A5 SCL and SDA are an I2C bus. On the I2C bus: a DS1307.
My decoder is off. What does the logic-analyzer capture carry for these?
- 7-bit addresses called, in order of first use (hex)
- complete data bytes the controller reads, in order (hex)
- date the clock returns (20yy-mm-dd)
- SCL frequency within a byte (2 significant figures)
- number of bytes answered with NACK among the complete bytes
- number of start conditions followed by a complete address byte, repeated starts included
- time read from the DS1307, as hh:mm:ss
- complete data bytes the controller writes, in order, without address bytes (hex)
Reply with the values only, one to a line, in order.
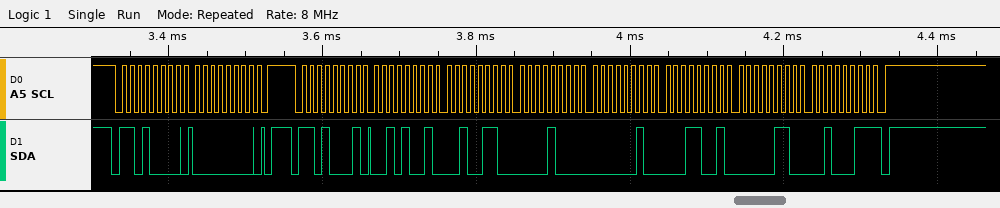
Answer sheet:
0x68
29 26 08 02 19 06 23
2023-06-19
100 kHz
1
2
08:26:29
00
